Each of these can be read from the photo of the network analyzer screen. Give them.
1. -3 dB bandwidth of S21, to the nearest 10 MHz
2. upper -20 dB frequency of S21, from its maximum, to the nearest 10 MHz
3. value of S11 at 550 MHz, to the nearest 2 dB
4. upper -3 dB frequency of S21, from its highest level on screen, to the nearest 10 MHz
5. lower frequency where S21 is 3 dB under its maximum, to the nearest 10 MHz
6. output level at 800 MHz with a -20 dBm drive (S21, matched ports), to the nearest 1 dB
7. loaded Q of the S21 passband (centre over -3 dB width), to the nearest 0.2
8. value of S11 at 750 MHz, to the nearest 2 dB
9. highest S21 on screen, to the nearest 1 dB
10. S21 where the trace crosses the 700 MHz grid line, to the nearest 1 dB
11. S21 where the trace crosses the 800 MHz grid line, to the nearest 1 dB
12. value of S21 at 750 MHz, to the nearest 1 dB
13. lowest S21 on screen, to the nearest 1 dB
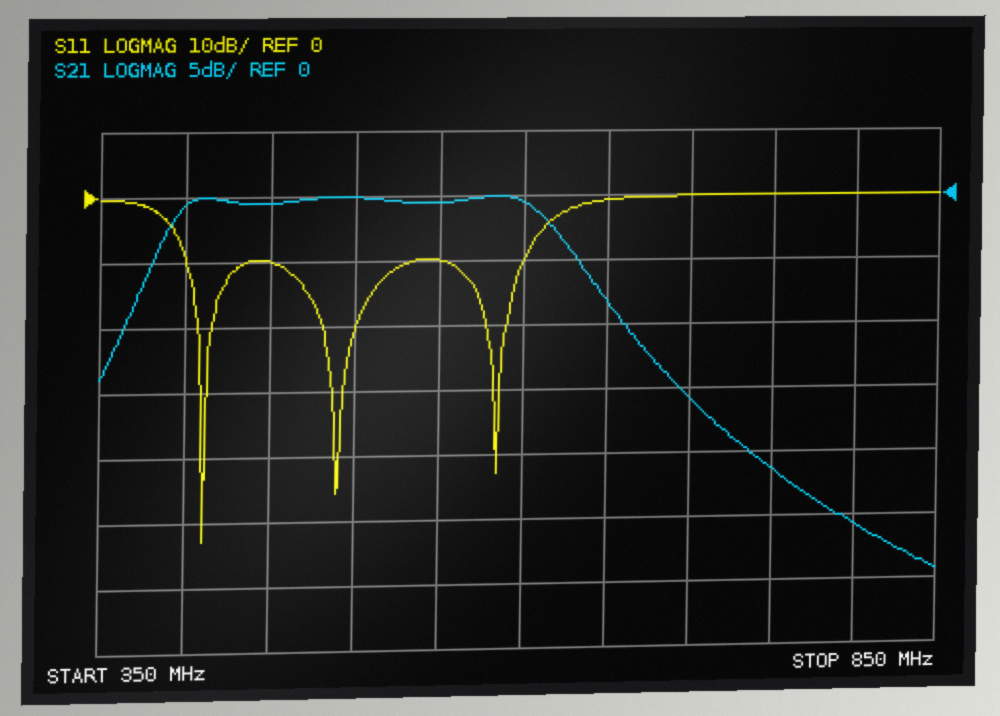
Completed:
230 MHz
740 MHz
-10 dB
620 MHz
390 MHz
-46 dBm
2.2
0 dB
0 dB
-16 dB
-26 dB
-21 dB
-29 dB
